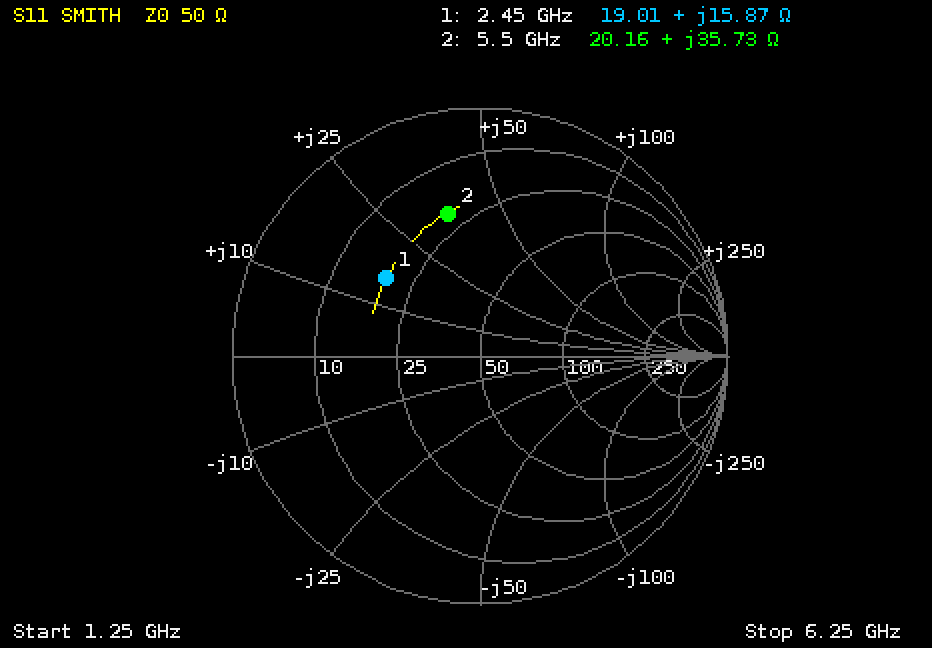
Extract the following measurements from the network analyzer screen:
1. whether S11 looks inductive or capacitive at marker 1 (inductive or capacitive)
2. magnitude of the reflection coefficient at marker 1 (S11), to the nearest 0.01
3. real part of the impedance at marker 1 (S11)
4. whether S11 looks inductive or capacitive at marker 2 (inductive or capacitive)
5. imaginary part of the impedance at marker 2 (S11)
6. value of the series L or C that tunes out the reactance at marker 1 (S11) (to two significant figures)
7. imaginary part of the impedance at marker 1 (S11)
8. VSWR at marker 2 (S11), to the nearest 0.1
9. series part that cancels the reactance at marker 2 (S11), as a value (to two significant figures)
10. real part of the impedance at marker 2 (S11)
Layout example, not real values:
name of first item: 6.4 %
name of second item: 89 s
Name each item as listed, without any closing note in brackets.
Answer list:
whether S11 looks inductive or capacitive at marker 1: inductive
magnitude of the reflection coefficient at marker 1 (S11), to the nearest 0.01: 0.49
real part of the impedance at marker 1: 19.01 Ω
whether S11 looks inductive or capacitive at marker 2: inductive
imaginary part of the impedance at marker 2: +35.73 Ω
value of the series L or C that tunes out the reactance at marker 1 (S11): 4.1 pF
imaginary part of the impedance at marker 1: +15.87 Ω
VSWR at marker 2 (S11), to the nearest 0.1: 3.9
series part that cancels the reactance at marker 2 (S11), as a value: 810 fF
real part of the impedance at marker 2: 20.16 Ω
